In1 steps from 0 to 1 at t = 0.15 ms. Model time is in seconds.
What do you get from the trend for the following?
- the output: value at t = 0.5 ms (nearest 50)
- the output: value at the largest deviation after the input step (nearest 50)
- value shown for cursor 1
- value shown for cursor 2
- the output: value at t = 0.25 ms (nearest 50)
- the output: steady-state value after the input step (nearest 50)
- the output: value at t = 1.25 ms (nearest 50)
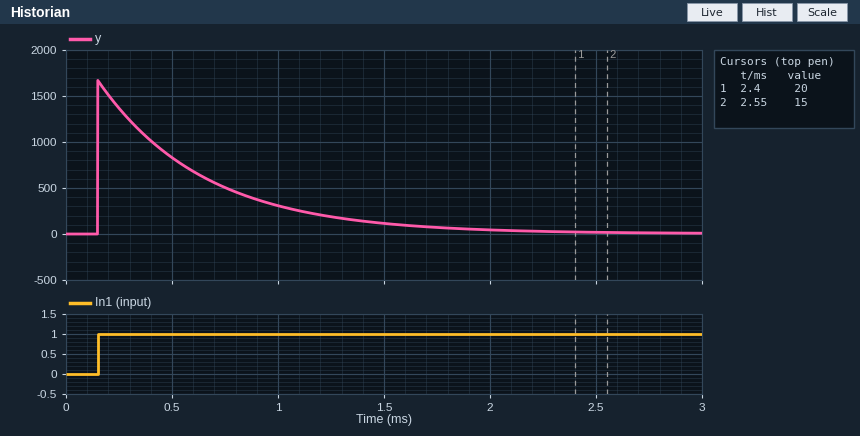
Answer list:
850
1650
20
15
1350
0
200
